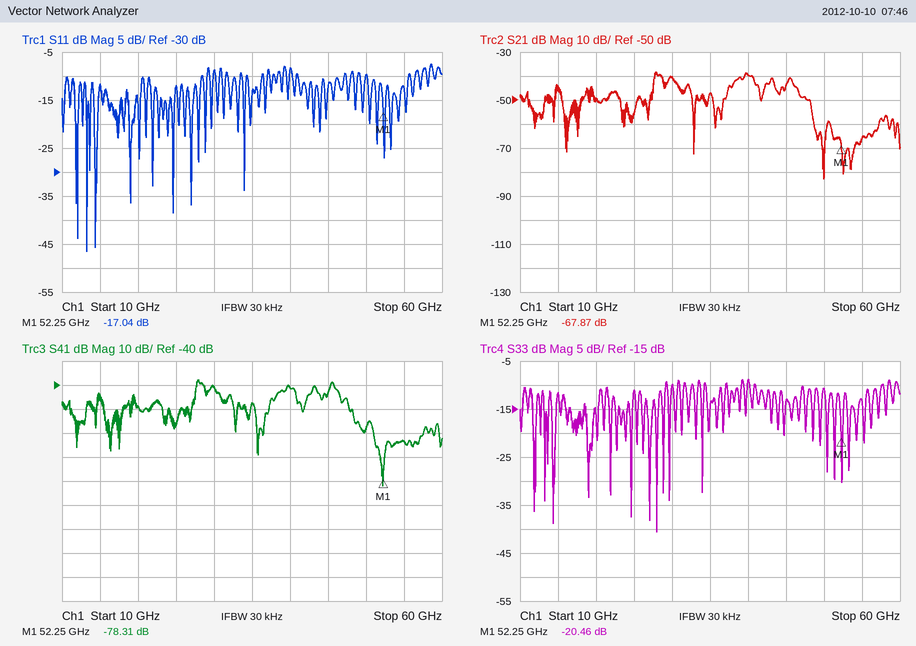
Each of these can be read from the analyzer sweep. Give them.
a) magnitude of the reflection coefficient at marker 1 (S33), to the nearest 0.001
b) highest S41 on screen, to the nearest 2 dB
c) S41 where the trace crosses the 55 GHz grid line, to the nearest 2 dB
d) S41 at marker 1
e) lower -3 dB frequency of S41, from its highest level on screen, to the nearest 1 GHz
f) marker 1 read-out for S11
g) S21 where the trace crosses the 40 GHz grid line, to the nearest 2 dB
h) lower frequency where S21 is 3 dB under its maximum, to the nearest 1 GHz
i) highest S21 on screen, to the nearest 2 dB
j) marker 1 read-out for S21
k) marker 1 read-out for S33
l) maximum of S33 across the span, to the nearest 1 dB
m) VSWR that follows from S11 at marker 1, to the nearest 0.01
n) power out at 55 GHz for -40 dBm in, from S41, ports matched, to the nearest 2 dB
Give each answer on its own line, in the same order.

0.095
-38 dB
-64 dB
-78.31 dB
28 GHz
-17.04 dB
-40 dB
28 GHz
-38 dB
-67.87 dB
-20.46 dB
-9 dB
1.33
-104 dBm
